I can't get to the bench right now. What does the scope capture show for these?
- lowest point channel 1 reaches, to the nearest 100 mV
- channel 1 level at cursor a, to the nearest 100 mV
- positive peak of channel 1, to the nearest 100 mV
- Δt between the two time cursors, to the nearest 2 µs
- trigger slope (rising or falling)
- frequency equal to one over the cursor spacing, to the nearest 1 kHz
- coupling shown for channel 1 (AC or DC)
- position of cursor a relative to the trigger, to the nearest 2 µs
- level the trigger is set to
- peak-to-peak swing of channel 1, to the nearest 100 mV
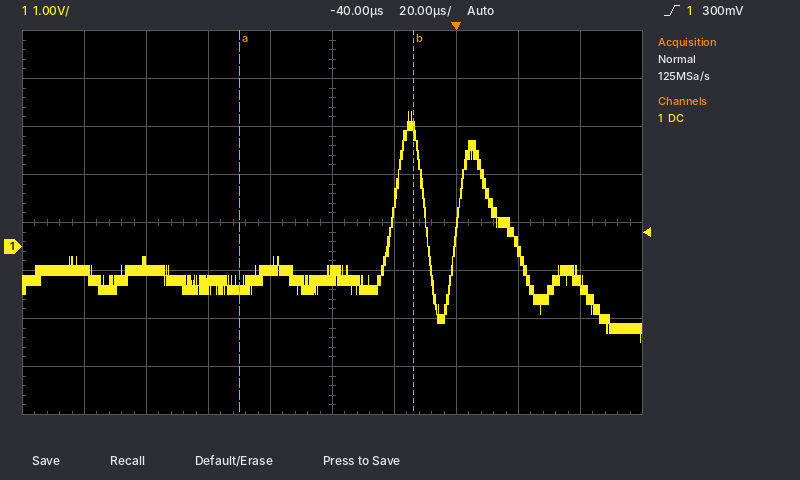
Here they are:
-2.0 V
-900 mV
2.8 V
56 µs
rising
18 kHz
DC
-70 µs
300 mV
4.8 V
